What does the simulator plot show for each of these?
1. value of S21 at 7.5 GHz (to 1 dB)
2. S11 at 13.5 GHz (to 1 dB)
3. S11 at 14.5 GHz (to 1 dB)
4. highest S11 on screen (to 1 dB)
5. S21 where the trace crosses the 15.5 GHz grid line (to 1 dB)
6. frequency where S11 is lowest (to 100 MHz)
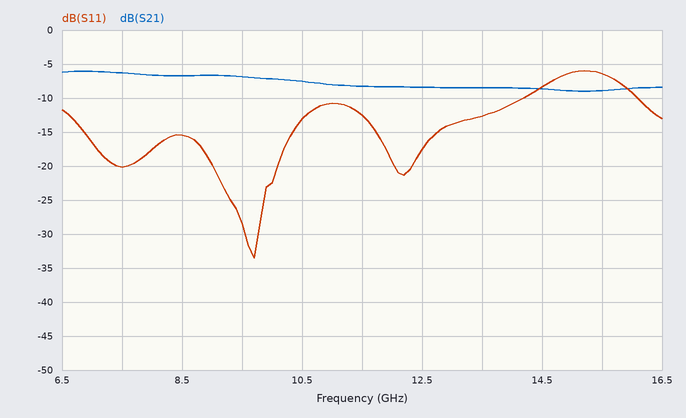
-6 dB
-13 dB
-8 dB
-6 dB
-9 dB
9.7 GHz
